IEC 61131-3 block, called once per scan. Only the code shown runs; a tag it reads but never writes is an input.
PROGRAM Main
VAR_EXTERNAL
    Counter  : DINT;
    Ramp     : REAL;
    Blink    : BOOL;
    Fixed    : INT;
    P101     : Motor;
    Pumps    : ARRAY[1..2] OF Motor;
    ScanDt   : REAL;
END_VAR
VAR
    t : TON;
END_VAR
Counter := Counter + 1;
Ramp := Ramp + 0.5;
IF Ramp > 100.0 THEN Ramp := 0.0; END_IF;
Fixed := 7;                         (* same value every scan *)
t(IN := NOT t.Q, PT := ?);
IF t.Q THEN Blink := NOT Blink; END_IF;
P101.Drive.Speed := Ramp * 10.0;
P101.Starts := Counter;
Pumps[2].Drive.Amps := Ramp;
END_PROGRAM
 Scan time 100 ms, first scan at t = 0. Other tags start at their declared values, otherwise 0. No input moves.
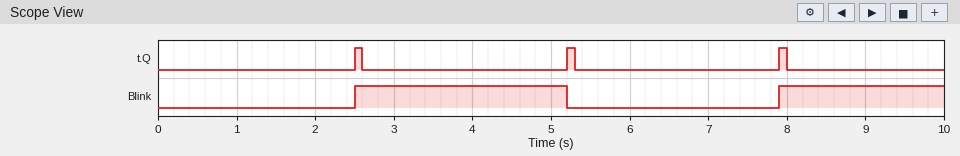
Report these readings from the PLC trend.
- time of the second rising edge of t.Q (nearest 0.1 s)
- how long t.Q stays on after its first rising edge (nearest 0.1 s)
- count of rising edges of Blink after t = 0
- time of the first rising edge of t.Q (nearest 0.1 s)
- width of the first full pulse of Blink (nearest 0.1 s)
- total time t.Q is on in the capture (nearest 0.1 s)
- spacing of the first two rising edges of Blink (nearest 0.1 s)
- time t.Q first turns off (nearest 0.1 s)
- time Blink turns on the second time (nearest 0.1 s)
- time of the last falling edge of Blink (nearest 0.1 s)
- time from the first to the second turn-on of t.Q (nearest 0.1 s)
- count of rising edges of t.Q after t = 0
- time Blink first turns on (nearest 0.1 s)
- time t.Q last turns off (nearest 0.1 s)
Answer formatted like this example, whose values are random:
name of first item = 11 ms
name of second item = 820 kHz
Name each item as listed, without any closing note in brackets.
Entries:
time of the second rising edge of t.Q = 5.2 s
how long t.Q stays on after its first rising edge = 0.1 s
count of rising edges of Blink after t = 0 = 2
time of the first rising edge of t.Q = 2.5 s
width of the first full pulse of Blink = 2.7 s
total time t.Q is on in the capture = 0.3 s
spacing of the first two rising edges of Blink = 5.4 s
time t.Q first turns off = 2.6 s
time Blink turns on the second time = 7.9 s
time of the last falling edge of Blink = 5.2 s
time from the first to the second turn-on of t.Q = 2.7 s
count of rising edges of t.Q after t = 0 = 3
time Blink first turns on = 2.5 s
time t.Q last turns off = 8.0 s
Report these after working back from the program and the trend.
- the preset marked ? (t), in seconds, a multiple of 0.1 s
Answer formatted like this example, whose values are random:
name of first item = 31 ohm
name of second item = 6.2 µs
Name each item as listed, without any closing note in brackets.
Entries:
the preset marked ? (t), in seconds, a multiple of 0.1 s = 2.5 s
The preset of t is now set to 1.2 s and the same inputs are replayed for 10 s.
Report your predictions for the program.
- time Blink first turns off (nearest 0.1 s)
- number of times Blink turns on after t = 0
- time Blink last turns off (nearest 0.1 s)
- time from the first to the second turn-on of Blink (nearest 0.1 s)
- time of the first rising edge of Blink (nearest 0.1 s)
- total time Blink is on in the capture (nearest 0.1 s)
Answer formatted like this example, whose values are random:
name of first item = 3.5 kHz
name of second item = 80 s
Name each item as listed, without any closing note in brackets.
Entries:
time Blink first turns off = 2.6 s
number of times Blink turns on after t = 0 = 4
time Blink last turns off = 8.2 s
time from the first to the second turn-on of Blink = 2.8 s
time of the first rising edge of Blink = 1.2 s
total time Blink is on in the capture = 4.6 s
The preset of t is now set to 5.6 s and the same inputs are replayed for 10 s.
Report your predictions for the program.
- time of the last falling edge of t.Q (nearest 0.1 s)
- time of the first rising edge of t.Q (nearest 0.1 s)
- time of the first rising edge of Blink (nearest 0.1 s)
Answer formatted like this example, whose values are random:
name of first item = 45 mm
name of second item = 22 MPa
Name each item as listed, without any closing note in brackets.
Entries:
time of the last falling edge of t.Q = 5.7 s
time of the first rising edge of t.Q = 5.6 s
time of the first rising edge of Blink = 5.6 s
